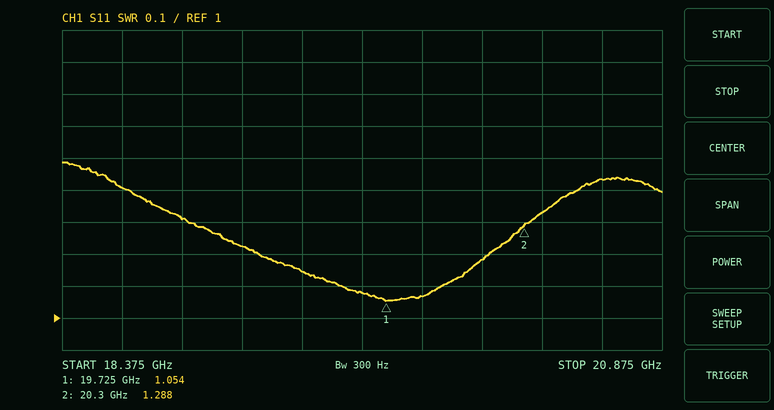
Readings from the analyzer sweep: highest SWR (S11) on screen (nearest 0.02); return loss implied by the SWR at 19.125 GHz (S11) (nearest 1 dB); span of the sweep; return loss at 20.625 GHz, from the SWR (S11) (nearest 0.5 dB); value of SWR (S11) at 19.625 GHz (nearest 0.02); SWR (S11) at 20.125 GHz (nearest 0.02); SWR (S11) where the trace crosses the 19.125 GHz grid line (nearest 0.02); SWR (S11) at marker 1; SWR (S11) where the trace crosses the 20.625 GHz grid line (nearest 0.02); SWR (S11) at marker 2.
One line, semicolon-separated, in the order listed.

1.48; 20 dB; 2.5 GHz; 15.0 dB; 1.08; 1.18; 1.22; 1.054; 1.44; 1.288
